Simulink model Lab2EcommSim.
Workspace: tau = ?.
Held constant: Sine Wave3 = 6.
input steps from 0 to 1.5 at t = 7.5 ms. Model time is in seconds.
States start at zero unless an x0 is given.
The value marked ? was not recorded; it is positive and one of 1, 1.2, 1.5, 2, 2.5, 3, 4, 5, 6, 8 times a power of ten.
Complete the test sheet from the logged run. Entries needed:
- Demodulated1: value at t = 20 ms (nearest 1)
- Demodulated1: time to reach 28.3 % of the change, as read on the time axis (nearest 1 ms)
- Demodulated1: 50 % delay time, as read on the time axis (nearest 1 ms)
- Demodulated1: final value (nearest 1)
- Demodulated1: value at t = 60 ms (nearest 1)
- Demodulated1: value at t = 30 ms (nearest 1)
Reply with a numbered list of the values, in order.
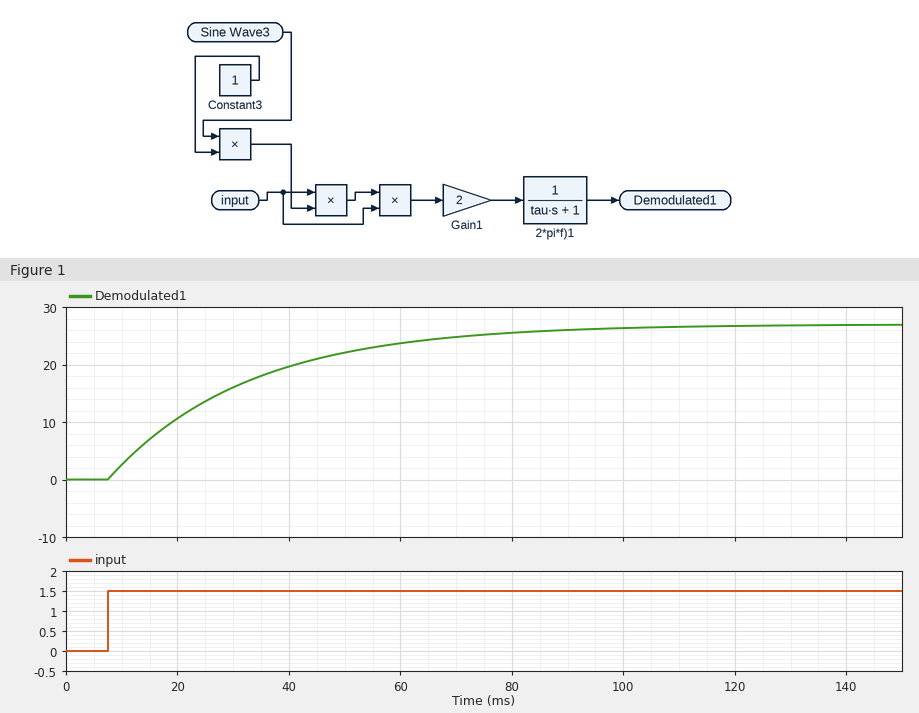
1. 11
2. 16 ms
3. 25 ms
4. 27
5. 24
6. 16
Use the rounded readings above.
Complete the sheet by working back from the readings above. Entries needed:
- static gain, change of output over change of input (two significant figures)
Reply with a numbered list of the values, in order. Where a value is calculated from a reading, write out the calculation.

1. (27 - 0) / (1.5 - 0) = 18
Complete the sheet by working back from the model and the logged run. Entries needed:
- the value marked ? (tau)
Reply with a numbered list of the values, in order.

1. 0.025
